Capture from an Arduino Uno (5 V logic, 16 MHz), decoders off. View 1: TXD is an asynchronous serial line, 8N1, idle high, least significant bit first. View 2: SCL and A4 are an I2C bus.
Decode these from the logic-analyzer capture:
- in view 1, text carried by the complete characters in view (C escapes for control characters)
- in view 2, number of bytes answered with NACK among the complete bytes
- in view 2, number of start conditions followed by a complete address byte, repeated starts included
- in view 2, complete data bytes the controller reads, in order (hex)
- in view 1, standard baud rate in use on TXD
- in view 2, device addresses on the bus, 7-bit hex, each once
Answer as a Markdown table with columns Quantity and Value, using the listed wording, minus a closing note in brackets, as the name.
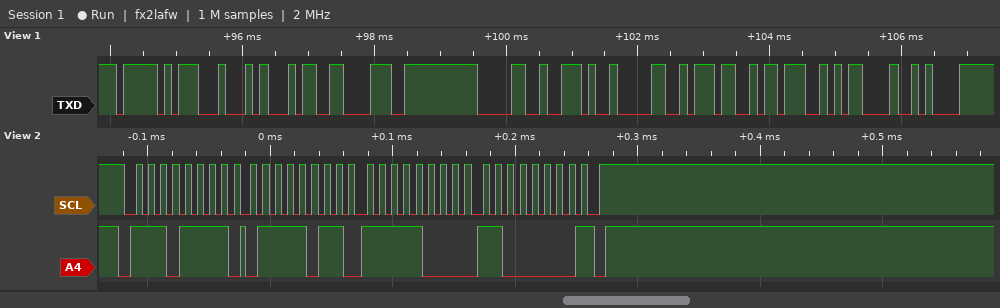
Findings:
| Quantity | Value |
|---|---|
| in view 1, text carried by the complete characters in view | "_D480.07;\r\n" |
| in view 2, number of bytes answered with NACK among the complete bytes | 1 |
| in view 2, number of start conditions followed by a complete address byte, repeated starts included | 1 |
| in view 2, complete data bytes the controller reads, in order | 7B F8 C0 |
| in view 1, standard baud rate in use on TXD | 9600 baud |
| in view 2, device addresses on the bus, 7-bit hex, each once | 0x77 |
